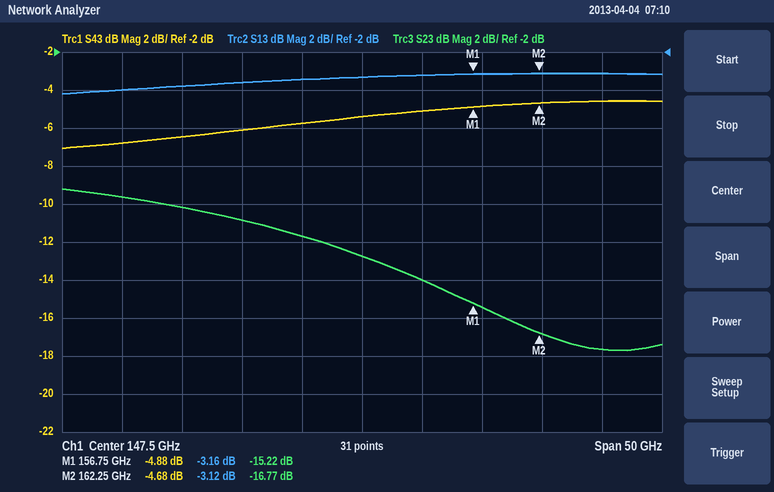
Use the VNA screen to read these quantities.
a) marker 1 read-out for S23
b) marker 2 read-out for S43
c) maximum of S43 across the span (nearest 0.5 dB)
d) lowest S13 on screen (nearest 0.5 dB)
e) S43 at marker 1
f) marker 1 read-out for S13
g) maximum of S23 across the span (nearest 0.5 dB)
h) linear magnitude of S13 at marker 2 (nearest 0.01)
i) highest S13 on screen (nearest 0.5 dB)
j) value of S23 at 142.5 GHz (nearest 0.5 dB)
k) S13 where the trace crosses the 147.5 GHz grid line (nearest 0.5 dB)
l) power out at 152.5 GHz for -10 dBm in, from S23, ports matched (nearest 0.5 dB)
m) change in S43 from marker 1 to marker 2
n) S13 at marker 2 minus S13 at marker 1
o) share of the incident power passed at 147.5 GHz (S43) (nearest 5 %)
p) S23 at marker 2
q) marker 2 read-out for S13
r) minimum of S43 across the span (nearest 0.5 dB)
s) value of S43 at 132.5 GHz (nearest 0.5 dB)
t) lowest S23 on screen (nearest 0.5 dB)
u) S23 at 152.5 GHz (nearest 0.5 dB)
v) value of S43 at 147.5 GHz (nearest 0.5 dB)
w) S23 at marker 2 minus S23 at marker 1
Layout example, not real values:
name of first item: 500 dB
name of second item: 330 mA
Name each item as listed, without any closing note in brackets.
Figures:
marker 1 read-out for S23: -15.22 dB
marker 2 read-out for S43: -4.68 dB
maximum of S43 across the span: -4.5 dB
lowest S13 on screen: -4.0 dB
S43 at marker 1: -4.88 dB
marker 1 read-out for S13: -3.16 dB
maximum of S23 across the span: -9.0 dB
linear magnitude of S13 at marker 2: 0.70
highest S13 on screen: -3.0 dB
value of S23 at 142.5 GHz: -11.5 dB
S13 where the trace crosses the 147.5 GHz grid line: -3.5 dB
power out at 152.5 GHz for -10 dBm in, from S23, ports matched: -24.0 dBm
change in S43 from marker 1 to marker 2: 0.20 dB
S13 at marker 2 minus S13 at marker 1: 0.04 dB
share of the incident power passed at 147.5 GHz (S43): 30 %
S23 at marker 2: -16.77 dB
marker 2 read-out for S13: -3.12 dB
minimum of S43 across the span: -7.0 dB
value of S43 at 132.5 GHz: -6.5 dB
lowest S23 on screen: -17.5 dB
S23 at 152.5 GHz: -14.0 dB
value of S43 at 147.5 GHz: -5.5 dB
S23 at marker 2 minus S23 at marker 1: -1.55 dB
